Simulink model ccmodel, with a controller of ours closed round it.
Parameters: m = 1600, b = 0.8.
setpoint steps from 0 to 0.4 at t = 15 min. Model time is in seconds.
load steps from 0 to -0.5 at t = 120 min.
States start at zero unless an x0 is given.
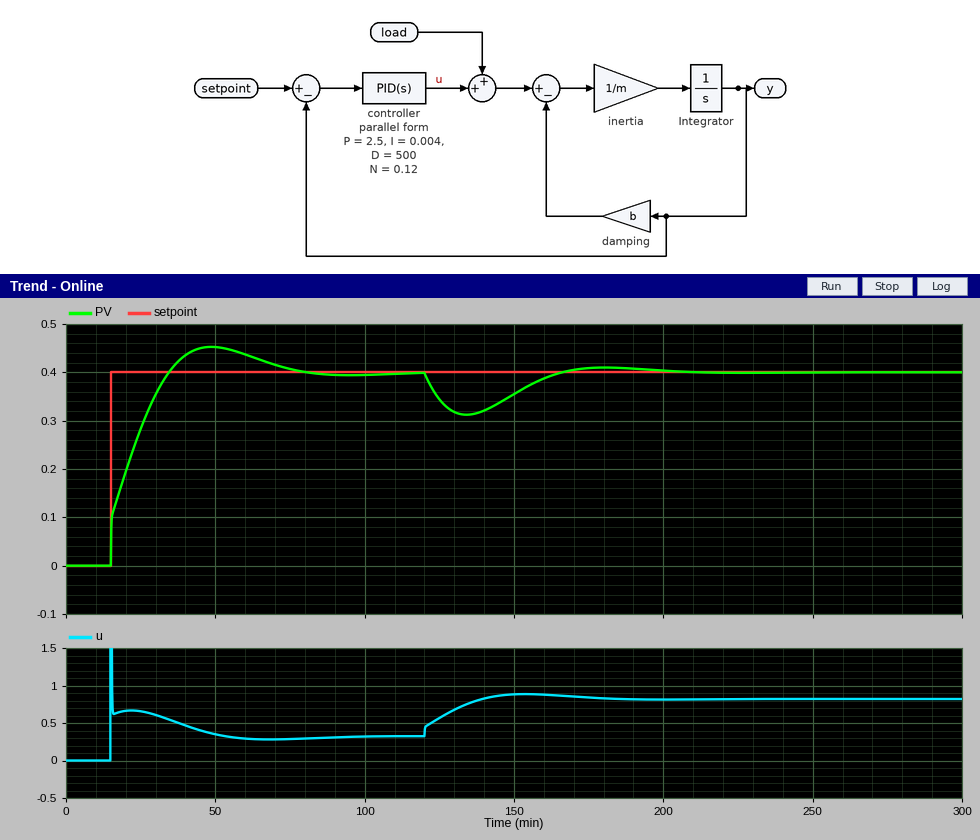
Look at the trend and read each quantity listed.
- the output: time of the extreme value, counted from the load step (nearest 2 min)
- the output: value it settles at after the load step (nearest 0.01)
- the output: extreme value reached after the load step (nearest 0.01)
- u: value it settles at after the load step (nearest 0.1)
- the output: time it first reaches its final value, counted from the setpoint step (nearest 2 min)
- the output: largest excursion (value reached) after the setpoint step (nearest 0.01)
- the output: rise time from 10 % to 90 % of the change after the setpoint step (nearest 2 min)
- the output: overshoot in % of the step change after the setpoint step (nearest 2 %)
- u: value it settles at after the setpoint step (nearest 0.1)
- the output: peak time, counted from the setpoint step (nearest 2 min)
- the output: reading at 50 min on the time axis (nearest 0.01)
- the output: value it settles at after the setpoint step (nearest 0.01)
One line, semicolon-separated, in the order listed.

14 min; 0.40; 0.31; 0.8; 20 min; 0.45; 16 min; 14 %; 0.3; 34 min; 0.45; 0.40
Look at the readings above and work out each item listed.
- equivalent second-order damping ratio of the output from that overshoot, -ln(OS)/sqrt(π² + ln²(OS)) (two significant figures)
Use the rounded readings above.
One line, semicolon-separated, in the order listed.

0.53
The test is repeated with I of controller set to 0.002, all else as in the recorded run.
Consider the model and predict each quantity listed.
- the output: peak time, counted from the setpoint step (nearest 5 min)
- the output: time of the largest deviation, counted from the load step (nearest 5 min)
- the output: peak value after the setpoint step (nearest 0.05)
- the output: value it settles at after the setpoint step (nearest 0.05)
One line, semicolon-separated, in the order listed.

50 min; 20 min; 0.40; 0.40
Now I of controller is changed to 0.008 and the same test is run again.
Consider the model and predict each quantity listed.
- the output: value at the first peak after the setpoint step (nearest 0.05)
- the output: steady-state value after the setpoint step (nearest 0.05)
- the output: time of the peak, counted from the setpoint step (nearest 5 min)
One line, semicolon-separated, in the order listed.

0.50; 0.40; 25 min
